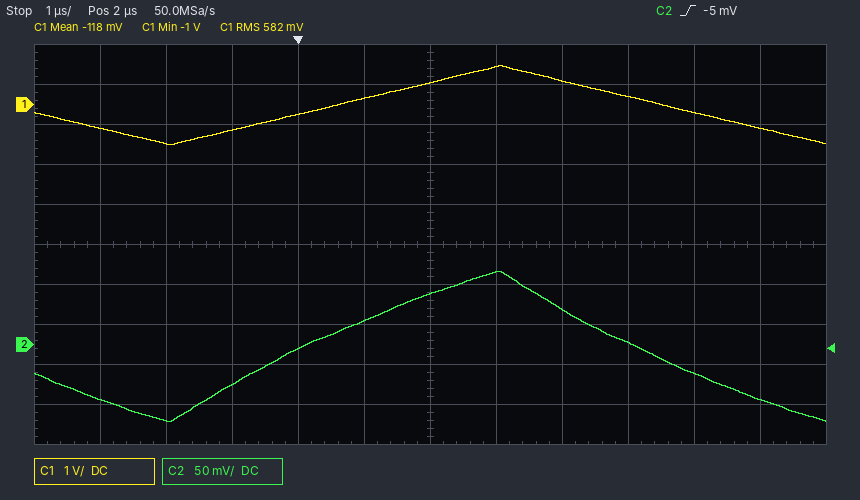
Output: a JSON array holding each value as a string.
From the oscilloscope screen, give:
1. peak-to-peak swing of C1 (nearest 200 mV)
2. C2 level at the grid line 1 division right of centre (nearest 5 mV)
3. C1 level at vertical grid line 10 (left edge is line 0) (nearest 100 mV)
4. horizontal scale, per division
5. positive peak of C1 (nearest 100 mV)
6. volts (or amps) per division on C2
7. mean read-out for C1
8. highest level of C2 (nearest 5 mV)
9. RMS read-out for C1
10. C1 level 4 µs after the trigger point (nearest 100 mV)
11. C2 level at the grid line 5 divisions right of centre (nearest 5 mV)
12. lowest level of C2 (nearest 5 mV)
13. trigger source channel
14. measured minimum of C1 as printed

["2.0 V", "90 mV", "-200 mV", "1 µs", "1.0 V", "50 mV", "-118 mV", "90 mV", "582 mV", "600 mV", "-70 mV", "-95 mV", "C2", "-1 V"]
